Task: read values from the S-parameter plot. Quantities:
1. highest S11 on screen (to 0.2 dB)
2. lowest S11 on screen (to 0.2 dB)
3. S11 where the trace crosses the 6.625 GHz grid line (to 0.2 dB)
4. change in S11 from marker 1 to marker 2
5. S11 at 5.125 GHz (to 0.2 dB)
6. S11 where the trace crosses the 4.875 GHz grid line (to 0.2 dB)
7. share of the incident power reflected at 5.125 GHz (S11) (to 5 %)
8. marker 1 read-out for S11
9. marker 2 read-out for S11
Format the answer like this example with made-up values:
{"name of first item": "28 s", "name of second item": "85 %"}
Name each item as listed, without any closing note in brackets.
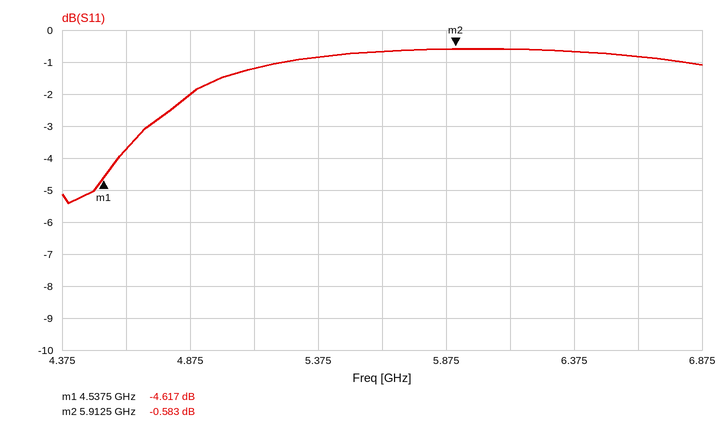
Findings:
{"highest S11 on screen": "-0.6 dB", "lowest S11 on screen": "-5.4 dB", "S11 where the trace crosses the 6.625 GHz grid line": "-0.8 dB", "change in S11 from marker 1 to marker 2": "4.034 dB", "S11 at 5.125 GHz": "-1.2 dB", "S11 where the trace crosses the 4.875 GHz grid line": "-2.0 dB", "share of the incident power reflected at 5.125 GHz (S11)": "75 %", "marker 1 read-out for S11": "-4.617 dB", "marker 2 read-out for S11": "-0.583 dB"}
